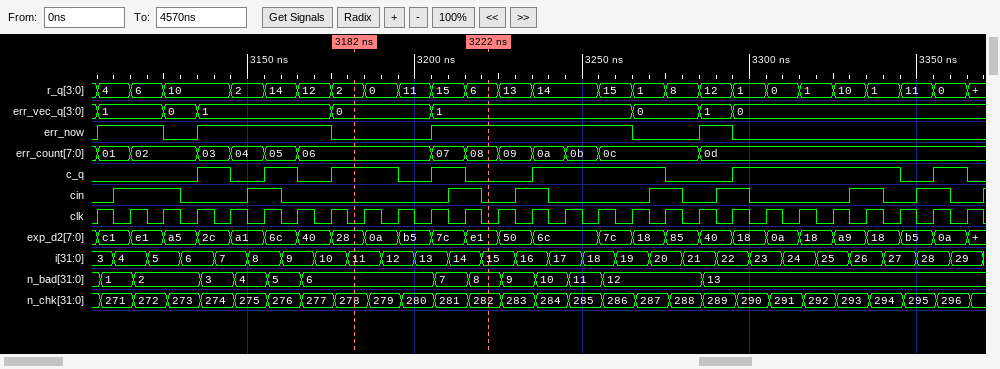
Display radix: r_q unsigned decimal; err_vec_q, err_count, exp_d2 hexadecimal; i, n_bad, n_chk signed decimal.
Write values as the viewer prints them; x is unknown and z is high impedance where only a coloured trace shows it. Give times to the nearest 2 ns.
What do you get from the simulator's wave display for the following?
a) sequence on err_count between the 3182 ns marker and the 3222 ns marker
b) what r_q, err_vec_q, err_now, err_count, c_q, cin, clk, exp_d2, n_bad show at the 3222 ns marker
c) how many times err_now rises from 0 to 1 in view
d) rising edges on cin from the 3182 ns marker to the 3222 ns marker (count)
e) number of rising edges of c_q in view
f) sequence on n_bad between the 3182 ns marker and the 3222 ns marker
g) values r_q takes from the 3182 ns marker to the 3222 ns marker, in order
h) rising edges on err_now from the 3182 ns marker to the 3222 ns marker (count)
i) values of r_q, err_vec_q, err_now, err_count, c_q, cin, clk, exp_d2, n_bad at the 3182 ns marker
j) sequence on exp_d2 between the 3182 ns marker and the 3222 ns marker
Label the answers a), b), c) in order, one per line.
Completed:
a) 06, 07, 08
b) r_q=6, err_vec_q=1, err_now=1, err_count=08, c_q=0, cin=0, clk=0, exp_d2=e1, n_bad=8
c) 4
d) 1
e) 7
f) 6, 7, 8
g) 2, 0, 11, 15, 6
h) 1
i) r_q=2, err_vec_q=0, err_now=0, err_count=06, c_q=1, cin=0, clk=0, exp_d2=28, n_bad=6
j) 28, 0a, b5, 7c, e1
